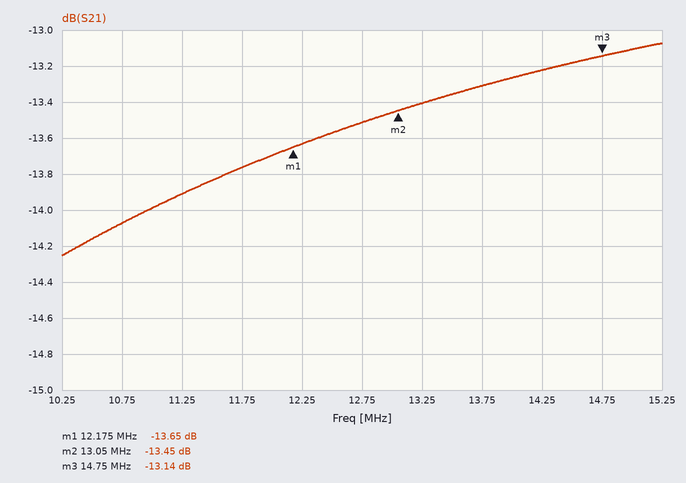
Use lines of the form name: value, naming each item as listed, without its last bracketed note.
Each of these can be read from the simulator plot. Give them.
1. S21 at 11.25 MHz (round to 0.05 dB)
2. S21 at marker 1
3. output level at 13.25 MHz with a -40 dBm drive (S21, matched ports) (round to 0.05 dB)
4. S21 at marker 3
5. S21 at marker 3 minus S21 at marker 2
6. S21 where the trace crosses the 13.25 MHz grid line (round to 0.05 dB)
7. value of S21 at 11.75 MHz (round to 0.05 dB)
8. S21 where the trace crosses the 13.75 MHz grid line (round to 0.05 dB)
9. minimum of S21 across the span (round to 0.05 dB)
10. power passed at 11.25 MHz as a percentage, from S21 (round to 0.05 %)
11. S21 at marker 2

S21 at 11.25 MHz: -13.90 dB
S21 at marker 1: -13.65 dB
output level at 13.25 MHz with a -40 dBm drive (S21, matched ports): -53.40 dBm
S21 at marker 3: -13.14 dB
S21 at marker 3 minus S21 at marker 2: 0.31 dB
S21 where the trace crosses the 13.25 MHz grid line: -13.40 dB
value of S21 at 11.75 MHz: -13.75 dB
S21 where the trace crosses the 13.75 MHz grid line: -13.30 dB
minimum of S21 across the span: -14.25 dB
power passed at 11.25 MHz as a percentage, from S21: 4.05 %
S21 at marker 2: -13.45 dB
